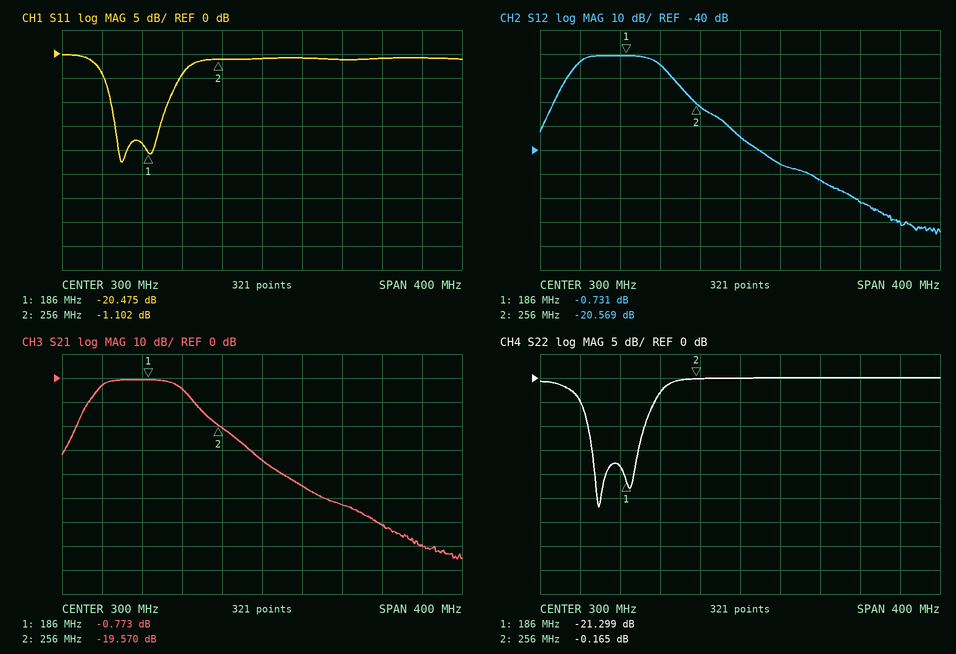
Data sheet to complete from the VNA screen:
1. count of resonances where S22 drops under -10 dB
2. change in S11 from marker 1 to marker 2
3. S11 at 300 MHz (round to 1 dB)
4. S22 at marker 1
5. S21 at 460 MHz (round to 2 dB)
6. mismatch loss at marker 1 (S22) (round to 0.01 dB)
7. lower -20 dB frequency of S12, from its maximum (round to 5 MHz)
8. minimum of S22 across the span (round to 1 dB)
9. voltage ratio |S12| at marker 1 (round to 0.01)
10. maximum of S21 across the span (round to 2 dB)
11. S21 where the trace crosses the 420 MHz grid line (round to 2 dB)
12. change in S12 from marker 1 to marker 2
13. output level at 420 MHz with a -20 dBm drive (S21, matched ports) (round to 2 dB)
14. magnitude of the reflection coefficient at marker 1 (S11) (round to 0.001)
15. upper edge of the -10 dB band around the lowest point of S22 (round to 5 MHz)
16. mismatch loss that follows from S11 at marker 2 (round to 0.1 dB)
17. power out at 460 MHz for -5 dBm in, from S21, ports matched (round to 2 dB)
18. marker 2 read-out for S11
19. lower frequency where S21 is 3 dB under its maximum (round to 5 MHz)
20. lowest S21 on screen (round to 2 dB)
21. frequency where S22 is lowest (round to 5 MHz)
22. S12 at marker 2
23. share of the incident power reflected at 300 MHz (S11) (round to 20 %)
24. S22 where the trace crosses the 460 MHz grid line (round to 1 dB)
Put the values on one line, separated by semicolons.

2; 19.373 dB; -1 dB; -21.299 dB; -70 dB; 0.03 dB; 115 MHz; -27 dB; 0.92; 0 dB; -62 dB; -19.838 dB; -82 dBm; 0.095; 205 MHz; 6.5 dB; -74 dBm; -1.102 dB; 140 MHz; -76 dB; 160 MHz; -20.569 dB; 80 %; 0 dB
